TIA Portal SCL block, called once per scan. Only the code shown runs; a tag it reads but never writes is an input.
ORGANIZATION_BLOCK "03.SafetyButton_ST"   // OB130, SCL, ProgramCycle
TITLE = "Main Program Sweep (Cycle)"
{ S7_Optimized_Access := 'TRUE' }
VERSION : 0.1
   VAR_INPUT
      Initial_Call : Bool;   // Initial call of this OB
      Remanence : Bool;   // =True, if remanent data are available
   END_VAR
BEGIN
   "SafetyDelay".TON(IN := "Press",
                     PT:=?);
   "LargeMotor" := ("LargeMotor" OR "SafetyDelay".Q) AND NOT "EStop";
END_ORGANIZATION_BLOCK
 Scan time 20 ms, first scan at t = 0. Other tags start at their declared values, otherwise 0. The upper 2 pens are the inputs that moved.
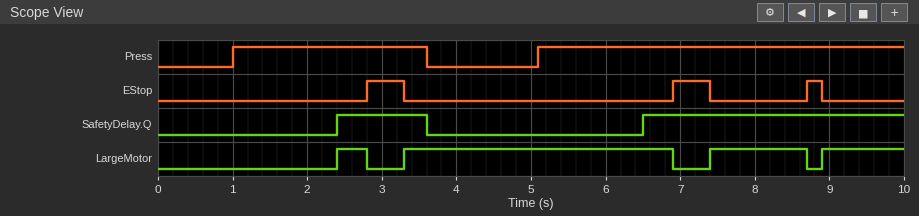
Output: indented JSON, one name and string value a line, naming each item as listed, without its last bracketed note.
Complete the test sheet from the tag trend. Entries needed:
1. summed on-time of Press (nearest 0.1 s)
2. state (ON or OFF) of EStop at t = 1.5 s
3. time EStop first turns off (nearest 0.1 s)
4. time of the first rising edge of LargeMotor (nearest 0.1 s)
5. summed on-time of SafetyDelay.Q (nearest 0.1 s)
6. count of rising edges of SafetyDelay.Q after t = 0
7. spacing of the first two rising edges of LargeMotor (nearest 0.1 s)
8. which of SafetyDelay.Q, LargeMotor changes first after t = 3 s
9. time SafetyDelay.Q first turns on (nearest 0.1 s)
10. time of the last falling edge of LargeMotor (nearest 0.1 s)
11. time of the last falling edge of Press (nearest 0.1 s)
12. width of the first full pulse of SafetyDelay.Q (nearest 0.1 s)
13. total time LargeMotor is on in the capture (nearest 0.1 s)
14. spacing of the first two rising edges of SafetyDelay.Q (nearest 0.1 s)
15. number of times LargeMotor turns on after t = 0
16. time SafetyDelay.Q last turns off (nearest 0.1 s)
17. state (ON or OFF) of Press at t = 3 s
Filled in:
{
  "summed on-time of Press": "7.5 s",
  "state (ON or OFF) of EStop at t = 1.5 s": "OFF",
  "time EStop first turns off": "3.3 s",
  "time of the first rising edge of LargeMotor": "2.4 s",
  "summed on-time of SafetyDelay.Q": "4.7 s",
  "count of rising edges of SafetyDelay.Q after t = 0": "2",
  "spacing of the first two rising edges of LargeMotor": "0.9 s",
  "which of SafetyDelay.Q, LargeMotor changes first after t = 3 s": "LargeMotor",
  "time SafetyDelay.Q first turns on": "2.4 s",
  "time of the last falling edge of LargeMotor": "8.7 s",
  "time of the last falling edge of Press": "3.6 s",
  "width of the first full pulse of SafetyDelay.Q": "1.2 s",
  "total time LargeMotor is on in the capture": "6.4 s",
  "spacing of the first two rising edges of SafetyDelay.Q": "4.1 s",
  "number of times LargeMotor turns on after t = 0": "4",
  "time SafetyDelay.Q last turns off": "3.6 s",
  "state (ON or OFF) of Press at t = 3 s": "ON"
}
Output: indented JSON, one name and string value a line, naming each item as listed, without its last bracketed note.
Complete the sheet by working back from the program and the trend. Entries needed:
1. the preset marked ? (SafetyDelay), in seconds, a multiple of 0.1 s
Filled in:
{
  "the preset marked ? (SafetyDelay), in seconds, a multiple of 0.1 s": "1.4 s"
}
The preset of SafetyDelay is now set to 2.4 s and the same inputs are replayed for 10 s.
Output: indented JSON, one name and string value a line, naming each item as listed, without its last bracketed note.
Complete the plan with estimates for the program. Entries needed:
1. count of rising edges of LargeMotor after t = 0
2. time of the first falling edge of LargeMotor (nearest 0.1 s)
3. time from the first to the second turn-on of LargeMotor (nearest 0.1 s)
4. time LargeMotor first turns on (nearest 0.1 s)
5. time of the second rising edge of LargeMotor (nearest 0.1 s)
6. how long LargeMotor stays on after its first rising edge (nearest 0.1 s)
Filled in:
{
  "count of rising edges of LargeMotor after t = 0": "3",
  "time of the first falling edge of LargeMotor": "6.9 s",
  "time from the first to the second turn-on of LargeMotor": "4.1 s",
  "time LargeMotor first turns on": "3.4 s",
  "time of the second rising edge of LargeMotor": "7.5 s",
  "how long LargeMotor stays on after its first rising edge": "3.5 s"
}
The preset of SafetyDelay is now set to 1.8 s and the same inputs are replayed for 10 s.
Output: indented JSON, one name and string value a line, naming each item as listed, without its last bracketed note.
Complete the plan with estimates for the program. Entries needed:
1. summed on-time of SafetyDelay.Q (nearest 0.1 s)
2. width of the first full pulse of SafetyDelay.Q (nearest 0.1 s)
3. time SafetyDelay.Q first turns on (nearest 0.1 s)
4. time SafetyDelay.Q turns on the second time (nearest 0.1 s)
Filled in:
{
  "summed on-time of SafetyDelay.Q": "3.9 s",
  "width of the first full pulse of SafetyDelay.Q": "0.8 s",
  "time SafetyDelay.Q first turns on": "2.8 s",
  "time SafetyDelay.Q turns on the second time": "6.9 s"
}
